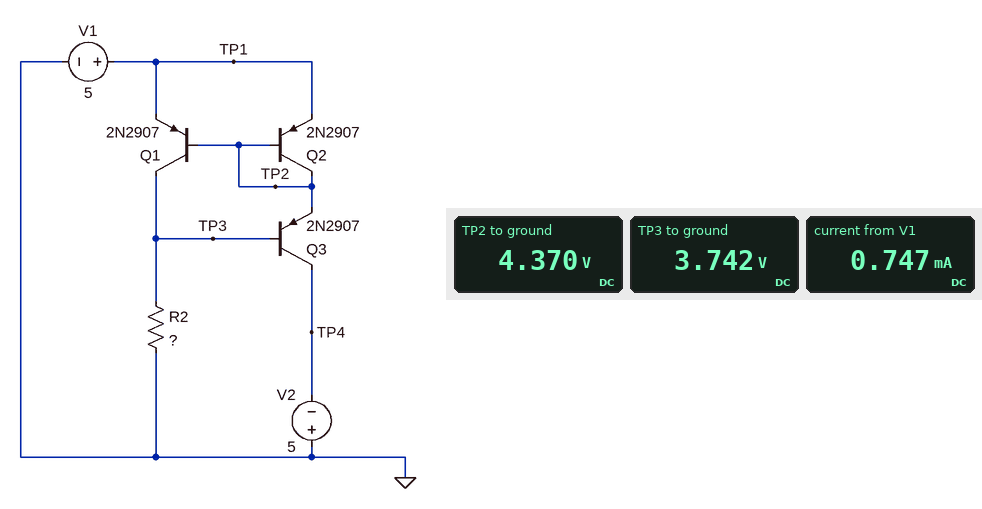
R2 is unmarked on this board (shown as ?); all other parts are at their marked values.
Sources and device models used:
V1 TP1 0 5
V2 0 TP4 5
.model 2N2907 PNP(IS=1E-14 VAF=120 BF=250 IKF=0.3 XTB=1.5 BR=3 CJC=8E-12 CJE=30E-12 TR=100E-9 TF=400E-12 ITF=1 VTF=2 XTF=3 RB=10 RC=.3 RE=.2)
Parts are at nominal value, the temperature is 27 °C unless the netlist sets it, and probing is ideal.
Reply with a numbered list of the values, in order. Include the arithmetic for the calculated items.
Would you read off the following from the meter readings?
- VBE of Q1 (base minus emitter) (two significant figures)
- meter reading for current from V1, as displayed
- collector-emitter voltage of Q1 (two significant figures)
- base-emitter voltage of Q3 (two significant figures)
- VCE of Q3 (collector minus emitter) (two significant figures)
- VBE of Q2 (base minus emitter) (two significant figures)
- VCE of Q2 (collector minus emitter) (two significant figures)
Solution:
1. 4.37 V - 5 V = -630 mV
2. 0.747 mA
3. 3.742 V - 5 V = -1.3 V
4. 3.742 V - 4.37 V = -630 mV
5. -5 V - 4.37 V = -9.4 V
6. 4.37 V - 5 V = -630 mV
7. 4.37 V - 5 V = -630 mV
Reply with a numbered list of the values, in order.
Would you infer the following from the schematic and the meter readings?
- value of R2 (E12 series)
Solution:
1. 10 kΩ
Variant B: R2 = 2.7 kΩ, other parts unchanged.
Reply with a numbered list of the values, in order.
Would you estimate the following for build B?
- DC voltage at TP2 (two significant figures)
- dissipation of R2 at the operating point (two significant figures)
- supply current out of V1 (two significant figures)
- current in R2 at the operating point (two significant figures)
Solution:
1. 4.3 V
2. 5.0 mW
3. 2.7 mA
4. 1.4 mA
